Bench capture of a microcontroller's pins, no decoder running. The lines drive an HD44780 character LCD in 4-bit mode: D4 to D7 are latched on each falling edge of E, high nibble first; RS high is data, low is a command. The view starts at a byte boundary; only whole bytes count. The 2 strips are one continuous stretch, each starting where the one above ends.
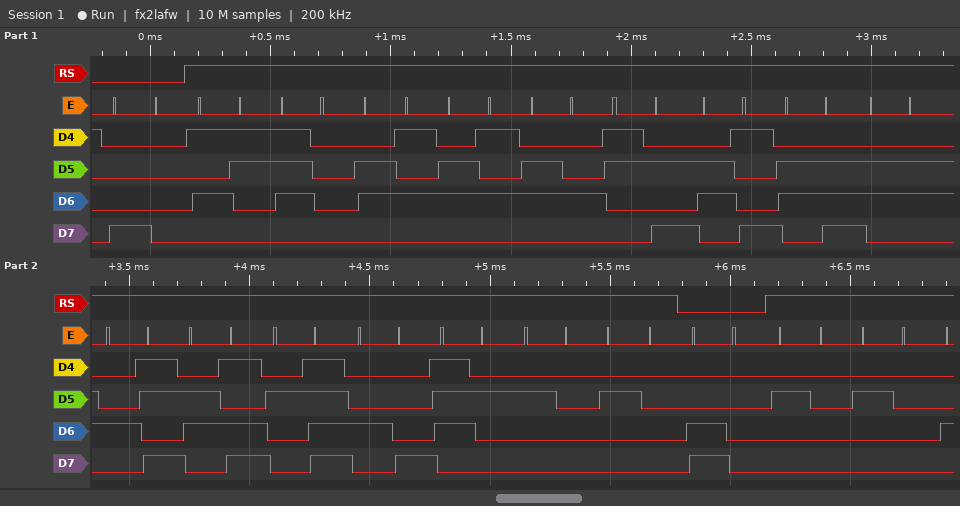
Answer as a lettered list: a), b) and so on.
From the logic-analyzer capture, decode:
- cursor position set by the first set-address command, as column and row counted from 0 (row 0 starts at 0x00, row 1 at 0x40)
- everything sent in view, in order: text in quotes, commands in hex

a) column 0, row 0
b) 0x80 "Speed:infKm/Hr  " 0xC0 "  "
